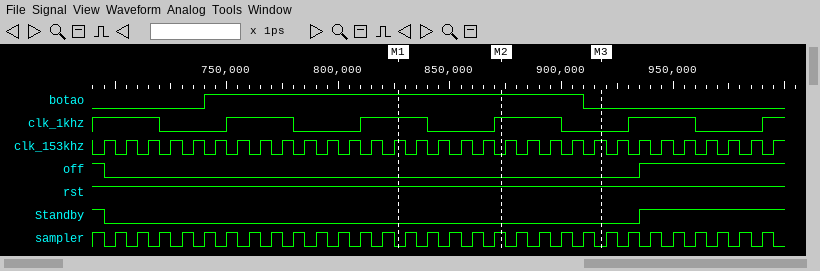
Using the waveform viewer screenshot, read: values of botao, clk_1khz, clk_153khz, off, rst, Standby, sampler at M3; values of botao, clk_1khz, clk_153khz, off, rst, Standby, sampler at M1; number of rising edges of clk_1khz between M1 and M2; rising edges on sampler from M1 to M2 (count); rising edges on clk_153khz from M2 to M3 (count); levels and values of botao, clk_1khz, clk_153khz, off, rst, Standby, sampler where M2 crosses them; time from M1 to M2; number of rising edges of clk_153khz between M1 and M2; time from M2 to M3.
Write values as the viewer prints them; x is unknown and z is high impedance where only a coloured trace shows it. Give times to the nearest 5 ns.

botao=0, clk_1khz=0, clk_153khz=1, off=0, rst=1, Standby=0, sampler=0
botao=1, clk_1khz=1, clk_153khz=1, off=0, rst=1, Standby=0, sampler=0
1
5
5
botao=1, clk_1khz=1, clk_153khz=0, off=0, rst=1, Standby=0, sampler=1
45 ns
4
45 ns
